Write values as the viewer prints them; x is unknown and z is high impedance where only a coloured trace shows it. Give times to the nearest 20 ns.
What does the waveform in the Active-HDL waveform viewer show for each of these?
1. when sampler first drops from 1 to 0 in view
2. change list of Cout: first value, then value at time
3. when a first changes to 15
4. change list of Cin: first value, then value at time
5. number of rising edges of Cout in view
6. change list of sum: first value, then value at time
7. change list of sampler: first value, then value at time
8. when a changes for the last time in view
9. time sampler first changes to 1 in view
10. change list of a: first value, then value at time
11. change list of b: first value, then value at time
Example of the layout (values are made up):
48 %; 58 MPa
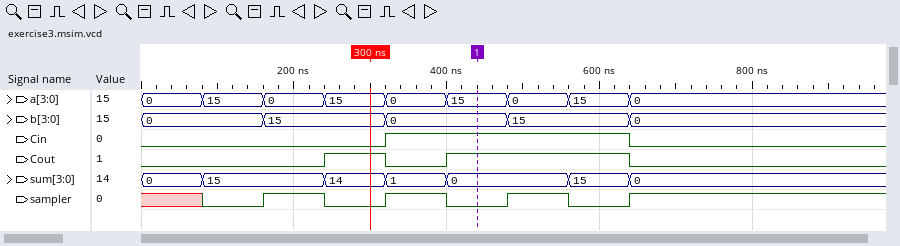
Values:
240 ns; 0, 1 at 240 ns, 0 at 320 ns, 1 at 400 ns, 0 at 640 ns; 80 ns; 0, 1 at 320 ns, 0 at 640 ns; 2; 0, 15 at 80 ns, 14 at 240 ns, 1 at 320 ns, 0 at 400 ns, 15 at 560 ns, 0 at 640 ns; x, 0 at 80 ns, 1 at 160 ns, 0 at 240 ns, 1 at 320 ns, 0 at 400 ns, 1 at 480 ns, 0 at 560 ns, 1 at 640 ns; 640 ns; 160 ns; 0, 15 at 80 ns, 0 at 160 ns, 15 at 240 ns, 0 at 320 ns, 15 at 400 ns, 0 at 480 ns, 15 at 560 ns, 0 at 640 ns; 0, 15 at 160 ns, 0 at 320 ns, 15 at 480 ns, 0 at 640 ns
